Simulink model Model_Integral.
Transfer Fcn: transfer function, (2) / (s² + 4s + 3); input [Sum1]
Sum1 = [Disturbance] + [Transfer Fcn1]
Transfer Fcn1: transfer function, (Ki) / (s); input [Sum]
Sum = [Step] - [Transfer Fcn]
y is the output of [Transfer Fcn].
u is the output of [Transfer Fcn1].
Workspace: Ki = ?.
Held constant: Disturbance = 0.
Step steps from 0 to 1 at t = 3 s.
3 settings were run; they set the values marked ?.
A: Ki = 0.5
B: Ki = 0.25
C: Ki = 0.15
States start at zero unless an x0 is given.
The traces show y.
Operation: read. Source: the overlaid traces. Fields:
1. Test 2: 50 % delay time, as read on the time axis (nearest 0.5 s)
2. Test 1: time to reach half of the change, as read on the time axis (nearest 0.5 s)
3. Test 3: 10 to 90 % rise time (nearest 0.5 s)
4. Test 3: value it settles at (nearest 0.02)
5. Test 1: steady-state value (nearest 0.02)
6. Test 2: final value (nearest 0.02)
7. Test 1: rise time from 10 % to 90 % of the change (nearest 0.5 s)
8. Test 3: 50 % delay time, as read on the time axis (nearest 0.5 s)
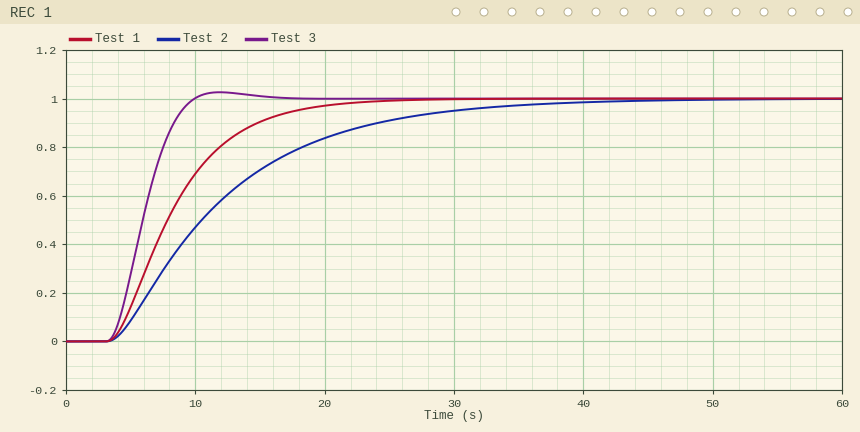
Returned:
10.5 s
8.0 s
4.0 s
1.00
1.00
1.00
10.0 s
6.0 s
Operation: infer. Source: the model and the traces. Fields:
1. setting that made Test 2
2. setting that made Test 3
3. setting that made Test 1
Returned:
C
A
B
